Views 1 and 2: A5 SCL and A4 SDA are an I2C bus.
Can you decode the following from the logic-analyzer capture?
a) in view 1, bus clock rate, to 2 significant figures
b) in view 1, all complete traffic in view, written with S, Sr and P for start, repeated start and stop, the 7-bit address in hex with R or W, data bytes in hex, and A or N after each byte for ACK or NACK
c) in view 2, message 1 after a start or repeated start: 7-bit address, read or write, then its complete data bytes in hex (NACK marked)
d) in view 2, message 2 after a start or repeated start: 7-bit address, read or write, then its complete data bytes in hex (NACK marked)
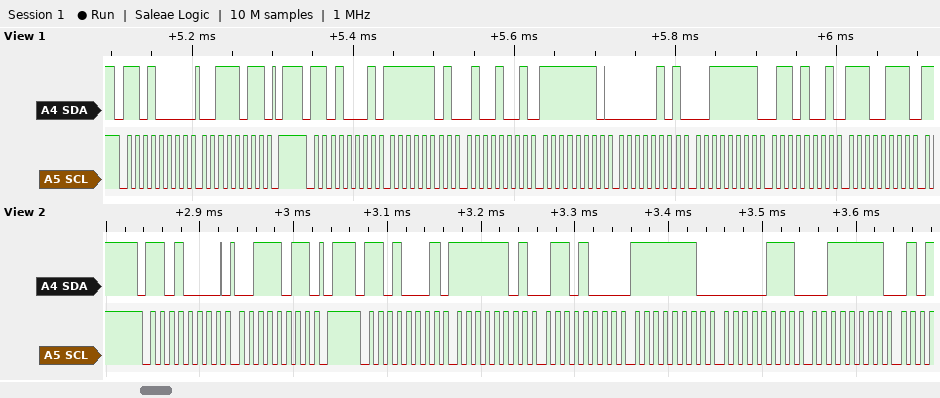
100 kHz
S 68W A 3B A P S 68R A FD A 49 A FE A 05 A 3F A 69 A E7 A
0x68 write: 3B
0x68 read: FD 68 FE 07 3F
